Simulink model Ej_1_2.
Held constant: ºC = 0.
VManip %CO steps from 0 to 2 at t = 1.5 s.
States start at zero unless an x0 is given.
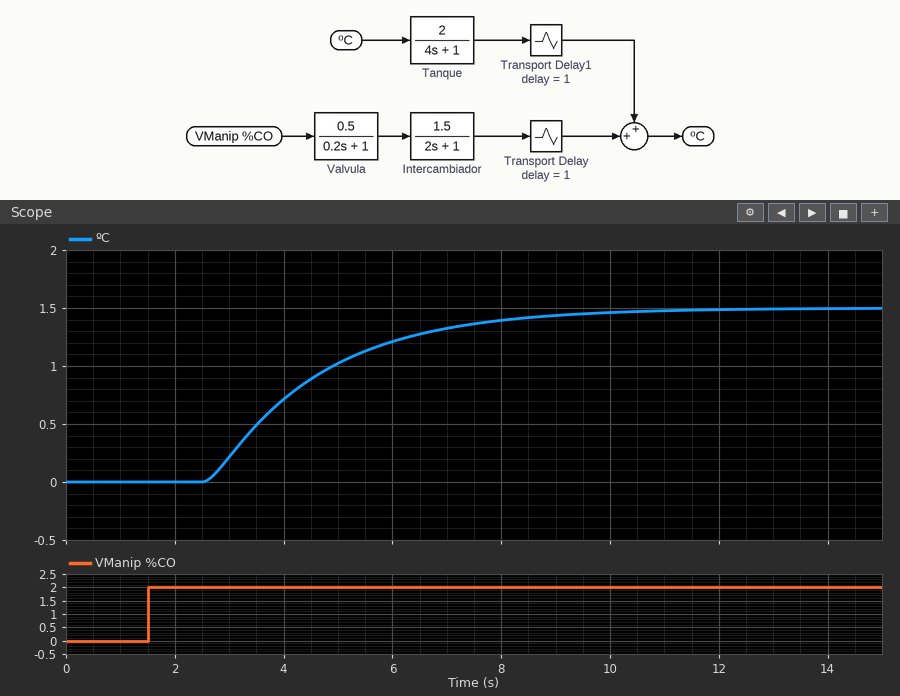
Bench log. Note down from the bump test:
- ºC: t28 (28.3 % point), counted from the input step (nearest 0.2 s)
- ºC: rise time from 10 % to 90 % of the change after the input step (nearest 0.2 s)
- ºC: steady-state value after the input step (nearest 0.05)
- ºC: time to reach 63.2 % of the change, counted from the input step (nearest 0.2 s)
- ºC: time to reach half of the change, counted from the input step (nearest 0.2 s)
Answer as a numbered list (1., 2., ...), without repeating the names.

1. 1.8 s
2. 4.4 s
3. 1.50
4. 3.2 s
5. 2.6 s
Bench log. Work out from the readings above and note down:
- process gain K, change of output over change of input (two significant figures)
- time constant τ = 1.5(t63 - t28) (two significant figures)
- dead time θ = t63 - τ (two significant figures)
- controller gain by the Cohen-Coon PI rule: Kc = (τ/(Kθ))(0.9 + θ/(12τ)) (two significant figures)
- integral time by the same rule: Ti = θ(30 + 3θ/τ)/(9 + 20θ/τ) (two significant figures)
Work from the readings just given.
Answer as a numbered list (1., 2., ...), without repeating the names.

1. 0.75
2. 2.1 s
3. 1.1 s
4. 2.4
5. 1.8 s
